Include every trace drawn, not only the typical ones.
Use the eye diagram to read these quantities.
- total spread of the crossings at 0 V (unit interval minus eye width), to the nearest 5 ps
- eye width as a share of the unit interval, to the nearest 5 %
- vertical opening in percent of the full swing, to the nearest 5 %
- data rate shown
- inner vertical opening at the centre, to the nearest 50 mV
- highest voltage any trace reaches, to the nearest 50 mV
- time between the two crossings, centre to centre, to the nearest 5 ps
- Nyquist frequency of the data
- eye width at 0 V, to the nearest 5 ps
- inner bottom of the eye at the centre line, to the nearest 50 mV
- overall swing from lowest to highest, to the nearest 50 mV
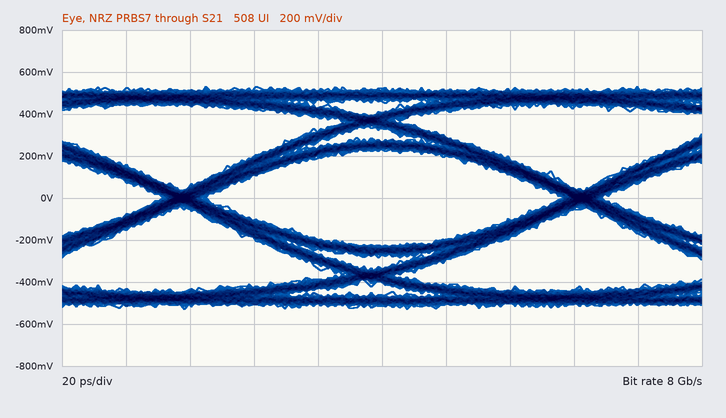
15 ps
90 %
45 %
8 Gb/s
450 mV
550 mV
125 ps
4 GHz
110 ps
-250 mV
1.05 V
